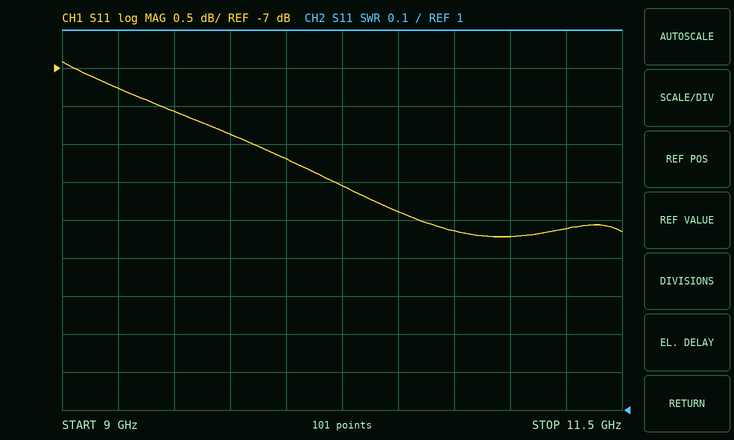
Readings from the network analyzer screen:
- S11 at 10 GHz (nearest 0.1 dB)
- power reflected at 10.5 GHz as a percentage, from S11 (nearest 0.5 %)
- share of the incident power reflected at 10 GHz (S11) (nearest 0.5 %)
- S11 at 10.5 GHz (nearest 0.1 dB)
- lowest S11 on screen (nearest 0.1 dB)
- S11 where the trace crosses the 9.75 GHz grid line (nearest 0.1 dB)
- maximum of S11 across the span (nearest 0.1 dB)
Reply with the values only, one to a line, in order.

-8.2 dB
13.0 %
15.0 %
-8.9 dB
-9.2 dB
-7.9 dB
-6.9 dB
